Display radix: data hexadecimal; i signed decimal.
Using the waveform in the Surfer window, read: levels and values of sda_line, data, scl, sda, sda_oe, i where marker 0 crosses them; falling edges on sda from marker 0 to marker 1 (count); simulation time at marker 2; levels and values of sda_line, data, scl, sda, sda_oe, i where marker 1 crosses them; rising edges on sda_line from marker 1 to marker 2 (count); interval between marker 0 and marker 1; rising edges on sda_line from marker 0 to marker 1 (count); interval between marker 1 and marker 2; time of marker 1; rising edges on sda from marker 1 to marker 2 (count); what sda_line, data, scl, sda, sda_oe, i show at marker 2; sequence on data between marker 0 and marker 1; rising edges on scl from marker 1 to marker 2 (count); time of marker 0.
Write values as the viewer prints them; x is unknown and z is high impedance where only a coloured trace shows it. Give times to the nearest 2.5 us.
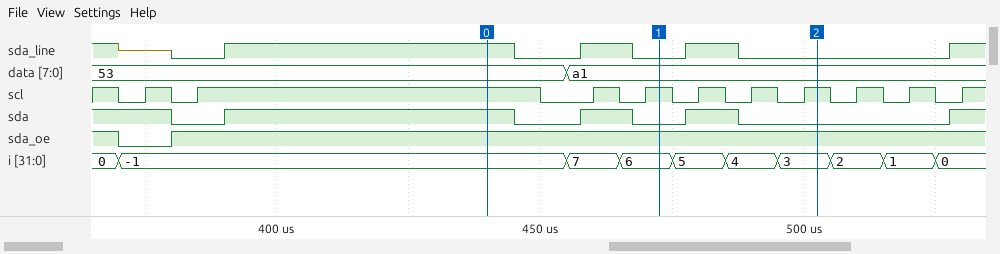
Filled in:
sda_line=1, data=53, scl=1, sda=1, sda_oe=1, i=-1
2
502.5 us
sda_line=0, data=a1, scl=1, sda=0, sda_oe=1, i=6
1
32.5 us
1
30 us
472.5 us
1
sda_line=0, data=a1, scl=1, sda=0, sda_oe=1, i=3
53, a1
3
440 us
